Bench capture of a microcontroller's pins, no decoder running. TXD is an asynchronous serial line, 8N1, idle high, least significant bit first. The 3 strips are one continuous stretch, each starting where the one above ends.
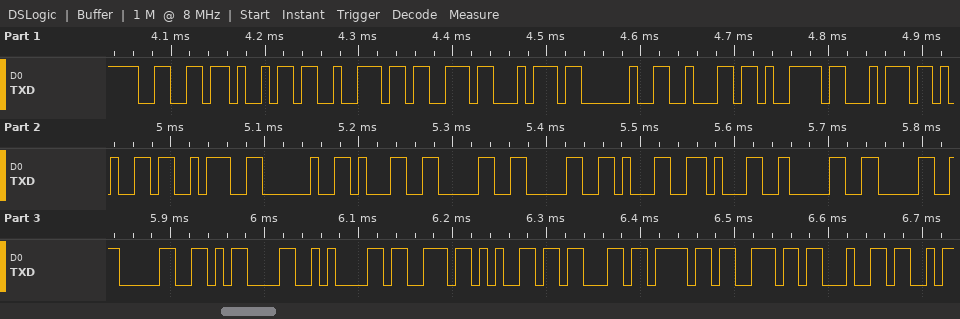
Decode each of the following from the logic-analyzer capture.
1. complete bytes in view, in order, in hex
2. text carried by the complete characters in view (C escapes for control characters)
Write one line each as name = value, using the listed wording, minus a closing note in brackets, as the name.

complete bytes in view, in order, in hex = 66 69 72 73 74 20 62 79 74 65 3A 20 31 30 30 31 31 30 30 30 0D 0A 73 65 63 6F 6E 64
text carried by the complete characters in view = "first byte: 10011000\r\nsecond"
